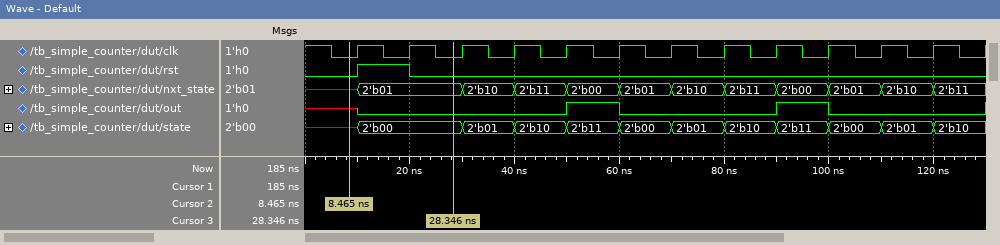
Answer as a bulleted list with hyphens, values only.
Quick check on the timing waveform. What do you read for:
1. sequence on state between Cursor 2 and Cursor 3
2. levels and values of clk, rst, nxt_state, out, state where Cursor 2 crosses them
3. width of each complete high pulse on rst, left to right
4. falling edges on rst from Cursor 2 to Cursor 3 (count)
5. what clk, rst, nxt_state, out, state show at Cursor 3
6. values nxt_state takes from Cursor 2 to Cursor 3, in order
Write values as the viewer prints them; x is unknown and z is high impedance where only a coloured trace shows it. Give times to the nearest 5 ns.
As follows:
- x, 2'b00
- clk=0, rst=0, nxt_state=x, out=x, state=x
- 10 ns
- 1
- clk=0, rst=0, nxt_state=2'b01, out=0, state=2'b00
- x, 2'b01
